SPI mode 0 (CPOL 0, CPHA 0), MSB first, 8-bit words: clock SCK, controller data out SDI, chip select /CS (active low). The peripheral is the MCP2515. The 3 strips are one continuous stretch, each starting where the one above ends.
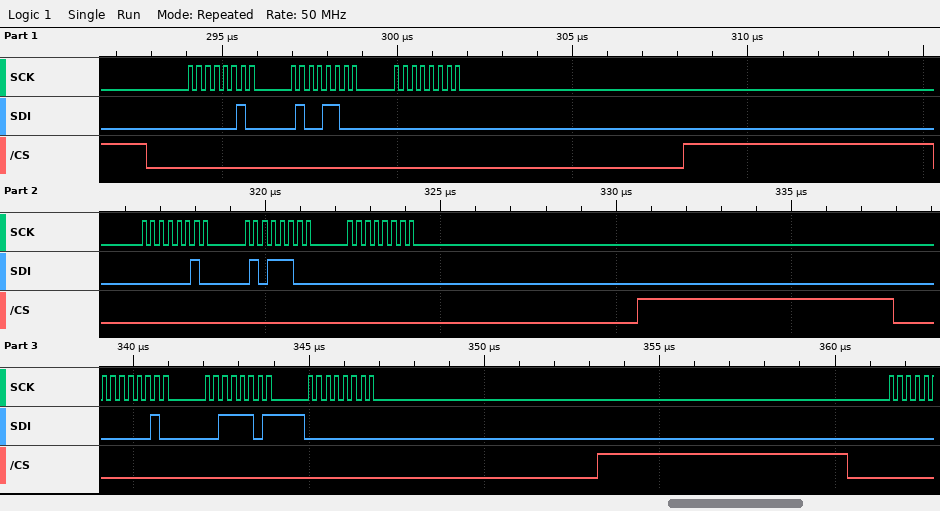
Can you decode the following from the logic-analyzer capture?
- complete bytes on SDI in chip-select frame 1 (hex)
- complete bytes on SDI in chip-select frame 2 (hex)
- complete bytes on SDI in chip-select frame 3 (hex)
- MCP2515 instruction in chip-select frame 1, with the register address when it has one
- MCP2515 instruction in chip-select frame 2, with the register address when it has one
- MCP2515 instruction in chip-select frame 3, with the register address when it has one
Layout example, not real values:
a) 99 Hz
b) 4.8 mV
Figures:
a) 02 4C 00
b) 02 5C 00
c) 02 3D 00
d) WRITE 0x4C
e) WRITE 0x5C
f) WRITE 0x3D
